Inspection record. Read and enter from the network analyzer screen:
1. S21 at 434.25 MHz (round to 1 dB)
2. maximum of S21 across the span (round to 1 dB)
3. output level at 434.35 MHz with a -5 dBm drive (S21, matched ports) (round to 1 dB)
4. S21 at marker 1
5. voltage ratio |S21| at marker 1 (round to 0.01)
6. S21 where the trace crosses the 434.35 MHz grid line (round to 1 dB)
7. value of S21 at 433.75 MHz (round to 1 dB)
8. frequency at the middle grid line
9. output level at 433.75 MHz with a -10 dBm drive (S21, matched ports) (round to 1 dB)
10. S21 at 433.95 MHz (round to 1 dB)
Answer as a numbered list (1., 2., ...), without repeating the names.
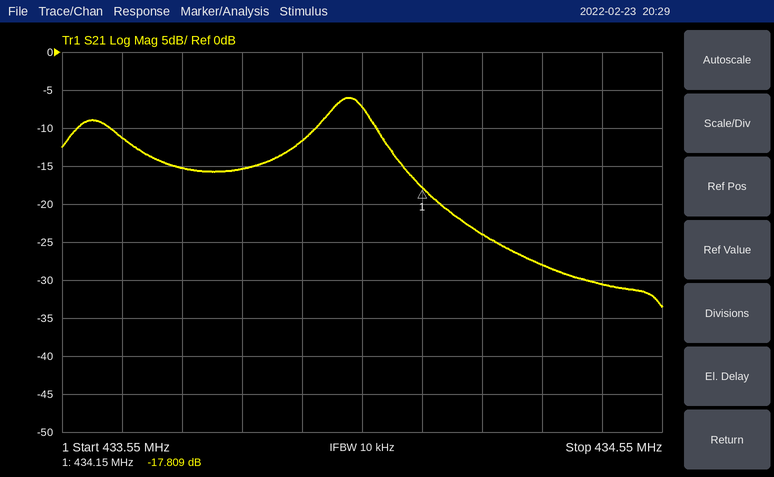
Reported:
1. -24 dB
2. -6 dB
3. -33 dBm
4. -17.809 dB
5. 0.13
6. -28 dB
7. -15 dB
8. 434.05 MHz
9. -25 dBm
10. -12 dB
